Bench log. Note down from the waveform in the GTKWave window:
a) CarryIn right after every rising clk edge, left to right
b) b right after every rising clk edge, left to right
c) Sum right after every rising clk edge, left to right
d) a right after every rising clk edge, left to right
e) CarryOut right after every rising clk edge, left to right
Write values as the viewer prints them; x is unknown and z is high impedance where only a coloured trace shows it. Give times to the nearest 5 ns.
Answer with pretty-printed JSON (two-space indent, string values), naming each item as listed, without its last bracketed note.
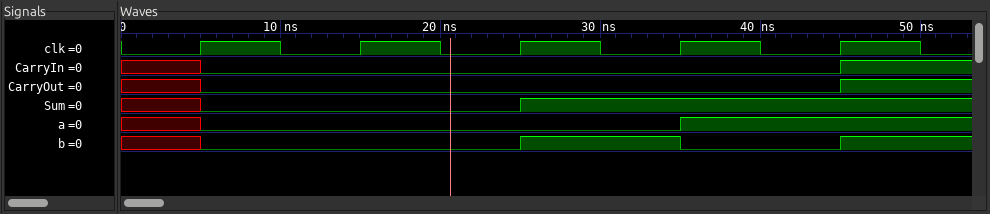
{
  "CarryIn right after every rising clk edge, left to right": "0 0 0 0 1",
  "b right after every rising clk edge, left to right": "0 0 1 0 1",
  "Sum right after every rising clk edge, left to right": "0 0 1 1 1",
  "a right after every rising clk edge, left to right": "0 0 0 1 1",
  "CarryOut right after every rising clk edge, left to right": "0 0 0 0 1"
}
